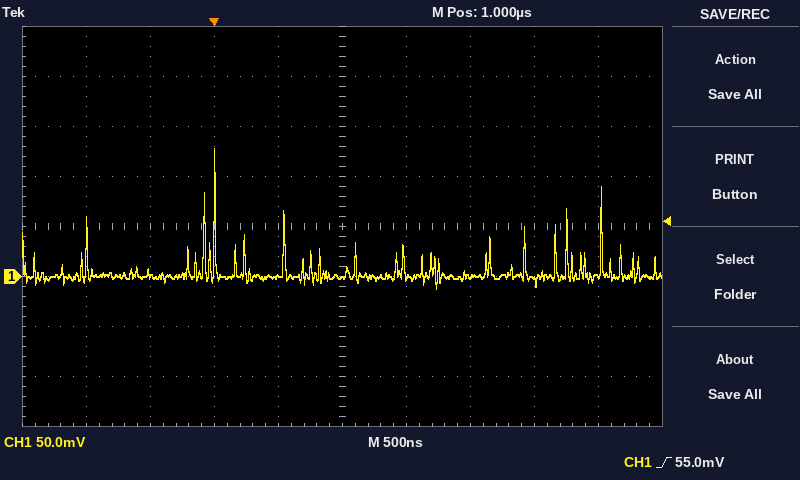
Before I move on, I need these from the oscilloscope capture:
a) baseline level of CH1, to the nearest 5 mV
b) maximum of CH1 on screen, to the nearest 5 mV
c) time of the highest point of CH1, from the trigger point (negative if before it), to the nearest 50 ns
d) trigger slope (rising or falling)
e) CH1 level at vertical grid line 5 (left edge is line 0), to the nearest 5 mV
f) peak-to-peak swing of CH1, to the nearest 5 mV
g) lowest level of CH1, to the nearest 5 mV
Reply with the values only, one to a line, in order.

0 mV
130 mV
0 ns
rising
0 mV
140 mV
-10 mV
